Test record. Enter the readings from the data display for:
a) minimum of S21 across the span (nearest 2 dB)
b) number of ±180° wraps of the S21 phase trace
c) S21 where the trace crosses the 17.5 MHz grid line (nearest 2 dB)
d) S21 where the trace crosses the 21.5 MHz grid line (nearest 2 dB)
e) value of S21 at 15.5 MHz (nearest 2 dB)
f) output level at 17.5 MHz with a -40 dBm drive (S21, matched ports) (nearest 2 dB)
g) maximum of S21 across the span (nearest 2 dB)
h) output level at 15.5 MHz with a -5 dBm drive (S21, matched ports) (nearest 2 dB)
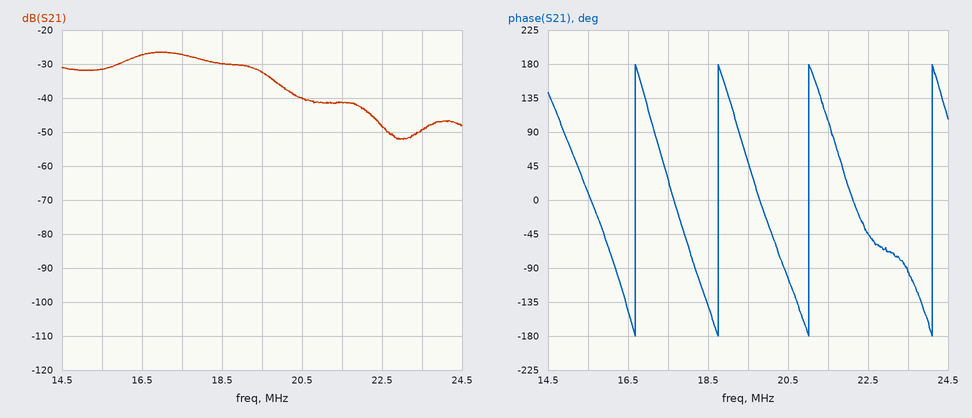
-52 dB
4
-28 dB
-42 dB
-32 dB
-68 dBm
-26 dB
-36 dBm
